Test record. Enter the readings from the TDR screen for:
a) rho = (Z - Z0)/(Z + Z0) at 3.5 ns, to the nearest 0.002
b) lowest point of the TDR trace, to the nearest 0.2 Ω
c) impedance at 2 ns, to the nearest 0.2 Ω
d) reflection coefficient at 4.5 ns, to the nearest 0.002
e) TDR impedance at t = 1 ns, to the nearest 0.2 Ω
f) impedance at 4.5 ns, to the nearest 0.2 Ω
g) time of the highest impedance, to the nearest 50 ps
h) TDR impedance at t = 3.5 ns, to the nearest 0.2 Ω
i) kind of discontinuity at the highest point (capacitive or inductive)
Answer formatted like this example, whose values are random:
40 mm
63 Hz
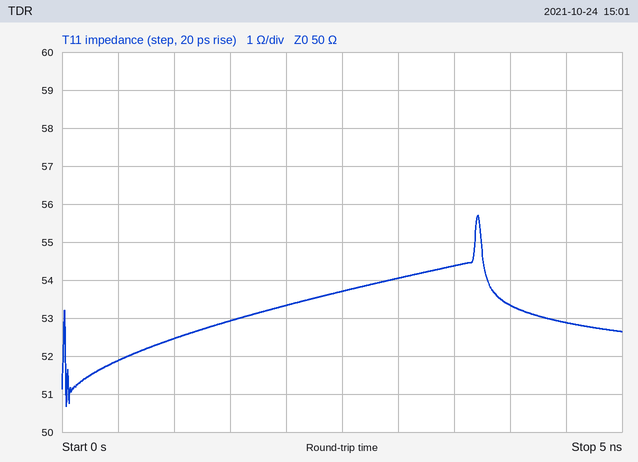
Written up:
+0.042
50.6 Ω
53.4 Ω
+0.028
52.4 Ω
52.8 Ω
3.70 ns
54.4 Ω
inductive
